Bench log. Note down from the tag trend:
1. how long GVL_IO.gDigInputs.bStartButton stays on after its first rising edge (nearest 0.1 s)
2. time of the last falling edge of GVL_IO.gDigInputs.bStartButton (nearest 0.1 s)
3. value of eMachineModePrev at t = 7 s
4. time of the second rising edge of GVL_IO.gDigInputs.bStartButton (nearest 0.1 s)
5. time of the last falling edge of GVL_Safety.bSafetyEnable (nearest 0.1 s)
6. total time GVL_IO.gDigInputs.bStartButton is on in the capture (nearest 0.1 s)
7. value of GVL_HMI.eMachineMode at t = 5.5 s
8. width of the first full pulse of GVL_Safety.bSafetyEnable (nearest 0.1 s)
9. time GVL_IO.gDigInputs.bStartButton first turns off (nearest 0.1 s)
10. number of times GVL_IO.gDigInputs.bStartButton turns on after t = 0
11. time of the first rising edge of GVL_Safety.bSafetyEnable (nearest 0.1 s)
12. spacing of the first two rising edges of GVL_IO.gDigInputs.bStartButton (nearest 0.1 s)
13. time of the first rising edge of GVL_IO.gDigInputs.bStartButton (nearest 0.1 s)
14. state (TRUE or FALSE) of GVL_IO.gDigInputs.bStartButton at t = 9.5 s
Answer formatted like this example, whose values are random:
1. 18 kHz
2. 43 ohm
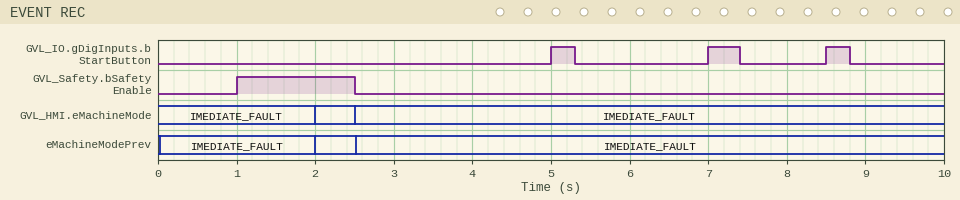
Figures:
1. 0.3 s
2. 8.8 s
3. IMEDIATE_FAULT
4. 7.0 s
5. 2.5 s
6. 1.0 s
7. IMEDIATE_FAULT
8. 1.5 s
9. 5.3 s
10. 3
11. 1.0 s
12. 2.0 s
13. 5.0 s
14. FALSE
